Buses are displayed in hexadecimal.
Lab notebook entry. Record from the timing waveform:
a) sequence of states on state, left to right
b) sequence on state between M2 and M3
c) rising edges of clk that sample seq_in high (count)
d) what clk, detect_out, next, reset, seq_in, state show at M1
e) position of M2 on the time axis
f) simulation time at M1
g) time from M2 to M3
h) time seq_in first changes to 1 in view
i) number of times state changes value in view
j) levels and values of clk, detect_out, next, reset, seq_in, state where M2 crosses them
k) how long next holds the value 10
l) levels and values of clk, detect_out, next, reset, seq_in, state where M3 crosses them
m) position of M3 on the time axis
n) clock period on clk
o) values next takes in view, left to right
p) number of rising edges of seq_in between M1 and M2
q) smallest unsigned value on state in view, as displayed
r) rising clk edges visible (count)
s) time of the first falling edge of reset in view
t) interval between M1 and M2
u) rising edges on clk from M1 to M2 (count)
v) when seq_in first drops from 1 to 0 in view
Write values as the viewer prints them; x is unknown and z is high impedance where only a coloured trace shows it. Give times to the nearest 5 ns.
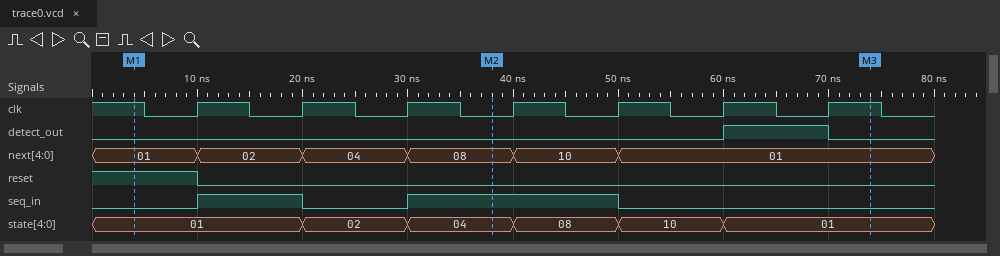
01, 02, 04, 08, 10, 01
04, 08, 10, 01
3
clk=1, detect_out=0, next=01, reset=1, seq_in=0, state=01
40 ns
5 ns
35 ns
10 ns
5
clk=0, detect_out=0, next=08, reset=0, seq_in=1, state=04
10 ns
clk=1, detect_out=0, next=01, reset=0, seq_in=0, state=01
75 ns
10 ns
01, 02, 04, 08, 10, 01
2
01
7
10 ns
35 ns
3
20 ns
